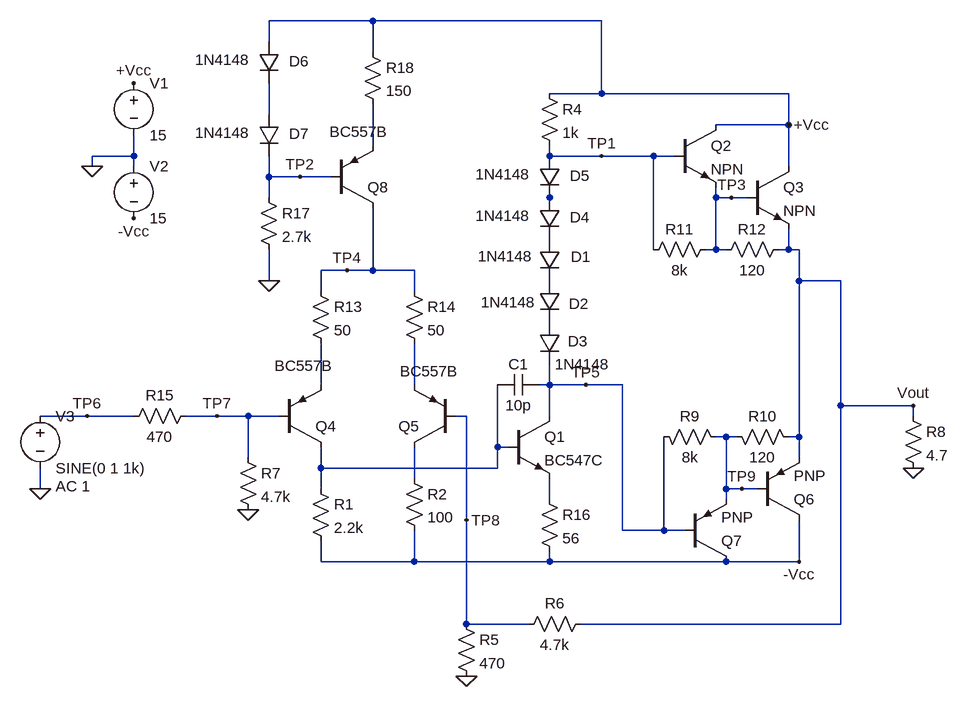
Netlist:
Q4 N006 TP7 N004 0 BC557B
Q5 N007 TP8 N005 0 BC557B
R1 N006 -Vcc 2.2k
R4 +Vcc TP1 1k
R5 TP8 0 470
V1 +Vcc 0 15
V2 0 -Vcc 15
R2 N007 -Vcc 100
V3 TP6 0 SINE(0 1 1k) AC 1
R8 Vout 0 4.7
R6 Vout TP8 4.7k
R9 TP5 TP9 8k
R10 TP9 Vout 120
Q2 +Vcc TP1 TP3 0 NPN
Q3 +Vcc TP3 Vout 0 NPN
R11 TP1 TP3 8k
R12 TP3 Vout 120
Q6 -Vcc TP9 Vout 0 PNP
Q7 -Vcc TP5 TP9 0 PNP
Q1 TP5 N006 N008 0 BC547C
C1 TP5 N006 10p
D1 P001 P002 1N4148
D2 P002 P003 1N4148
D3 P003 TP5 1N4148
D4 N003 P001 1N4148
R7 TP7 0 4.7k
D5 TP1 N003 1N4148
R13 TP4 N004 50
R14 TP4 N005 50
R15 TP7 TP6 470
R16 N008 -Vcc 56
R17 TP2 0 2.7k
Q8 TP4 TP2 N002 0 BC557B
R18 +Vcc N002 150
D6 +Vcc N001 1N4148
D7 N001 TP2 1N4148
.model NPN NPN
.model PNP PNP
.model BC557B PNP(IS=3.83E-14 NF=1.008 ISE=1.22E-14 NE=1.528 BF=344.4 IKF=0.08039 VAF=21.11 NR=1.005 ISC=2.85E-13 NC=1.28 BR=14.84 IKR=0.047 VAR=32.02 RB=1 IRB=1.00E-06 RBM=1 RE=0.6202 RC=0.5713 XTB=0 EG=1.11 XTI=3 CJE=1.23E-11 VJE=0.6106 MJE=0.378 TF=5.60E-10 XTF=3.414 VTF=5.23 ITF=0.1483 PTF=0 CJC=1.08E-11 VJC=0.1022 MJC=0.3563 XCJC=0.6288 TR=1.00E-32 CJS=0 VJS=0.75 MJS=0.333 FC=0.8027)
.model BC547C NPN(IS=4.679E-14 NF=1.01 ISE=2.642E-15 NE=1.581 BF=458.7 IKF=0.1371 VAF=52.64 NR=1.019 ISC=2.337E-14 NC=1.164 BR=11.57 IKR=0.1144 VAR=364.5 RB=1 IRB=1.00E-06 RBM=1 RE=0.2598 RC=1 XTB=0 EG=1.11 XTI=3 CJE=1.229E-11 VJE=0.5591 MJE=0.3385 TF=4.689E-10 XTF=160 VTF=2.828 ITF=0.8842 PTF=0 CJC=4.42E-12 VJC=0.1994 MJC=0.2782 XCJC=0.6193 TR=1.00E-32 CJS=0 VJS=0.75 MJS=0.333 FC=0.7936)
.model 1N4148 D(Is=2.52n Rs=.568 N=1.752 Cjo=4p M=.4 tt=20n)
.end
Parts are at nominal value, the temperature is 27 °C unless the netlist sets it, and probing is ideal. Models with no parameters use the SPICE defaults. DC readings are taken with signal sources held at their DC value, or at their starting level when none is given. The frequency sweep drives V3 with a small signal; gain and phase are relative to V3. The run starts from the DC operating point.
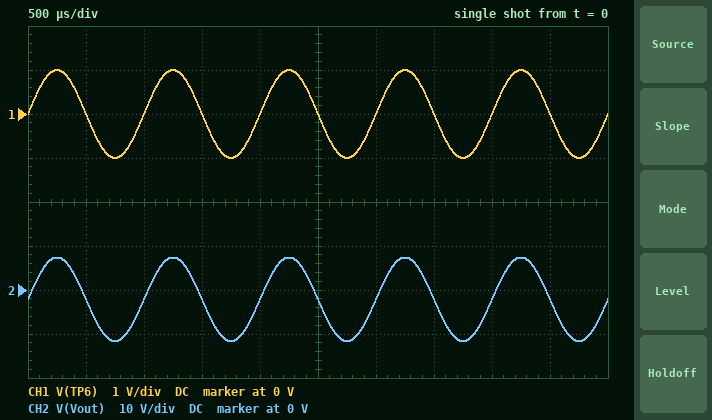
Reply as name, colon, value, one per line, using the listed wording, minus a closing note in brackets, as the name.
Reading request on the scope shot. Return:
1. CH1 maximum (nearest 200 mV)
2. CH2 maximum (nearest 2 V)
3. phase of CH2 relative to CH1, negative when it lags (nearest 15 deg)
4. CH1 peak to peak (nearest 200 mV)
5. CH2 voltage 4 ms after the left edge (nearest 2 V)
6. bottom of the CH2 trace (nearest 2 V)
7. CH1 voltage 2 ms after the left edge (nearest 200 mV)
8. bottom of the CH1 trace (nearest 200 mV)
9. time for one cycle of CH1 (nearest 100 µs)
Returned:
CH1 maximum: 1.0 V
CH2 maximum: 8 V
phase of CH2 relative to CH1, negative when it lags: 0 deg
CH1 peak to peak: 2.0 V
CH2 voltage 4 ms after the left edge: -2 V
bottom of the CH2 trace: -12 V
CH1 voltage 2 ms after the left edge: 0 V
bottom of the CH1 trace: -1.0 V
time for one cycle of CH1: 1.0 ms
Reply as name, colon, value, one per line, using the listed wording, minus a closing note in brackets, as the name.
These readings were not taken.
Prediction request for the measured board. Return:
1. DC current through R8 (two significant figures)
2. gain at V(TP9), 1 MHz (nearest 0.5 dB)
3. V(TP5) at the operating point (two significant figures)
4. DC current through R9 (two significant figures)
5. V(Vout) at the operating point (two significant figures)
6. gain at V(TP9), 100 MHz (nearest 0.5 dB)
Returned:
DC current through R8: 450 mA
gain at V(TP9), 1 MHz: 19.5 dB
V(TP5) at the operating point: -3.9 V
DC current through R9: 110 µA
V(Vout) at the operating point: -2.1 V
gain at V(TP9), 100 MHz: -14.5 dB
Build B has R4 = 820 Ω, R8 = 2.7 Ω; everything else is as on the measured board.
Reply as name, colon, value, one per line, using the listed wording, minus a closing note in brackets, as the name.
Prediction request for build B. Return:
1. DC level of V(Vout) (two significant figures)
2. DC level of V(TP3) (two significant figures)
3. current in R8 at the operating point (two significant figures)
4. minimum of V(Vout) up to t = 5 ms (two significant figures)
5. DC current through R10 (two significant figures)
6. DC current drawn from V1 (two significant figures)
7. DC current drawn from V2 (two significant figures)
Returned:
DC level of V(Vout): -2.0 V
DC level of V(TP3): -1.0 V
current in R8 at the operating point: 730 mA
minimum of V(Vout) up to t = 5 ms: -11 V
DC current through R10: 8.1 mA
DC current drawn from V1: 1.1 A
DC current drawn from V2: 1.8 A
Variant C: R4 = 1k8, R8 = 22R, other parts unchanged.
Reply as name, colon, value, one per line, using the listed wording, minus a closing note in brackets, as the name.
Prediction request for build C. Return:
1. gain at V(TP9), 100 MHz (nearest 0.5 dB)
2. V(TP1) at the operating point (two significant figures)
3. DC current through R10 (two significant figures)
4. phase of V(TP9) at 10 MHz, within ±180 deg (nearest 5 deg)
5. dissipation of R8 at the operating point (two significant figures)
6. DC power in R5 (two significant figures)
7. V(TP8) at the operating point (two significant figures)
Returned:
gain at V(TP9), 100 MHz: -15.0 dB
V(TP1) at the operating point: -750 mV
DC current through R10: 7.5 mA
phase of V(TP9) at 10 MHz, within ±180 deg: -90 deg
dissipation of R8 at the operating point: 270 mW
DC power in R5: 100 µW
V(TP8) at the operating point: -220 mV
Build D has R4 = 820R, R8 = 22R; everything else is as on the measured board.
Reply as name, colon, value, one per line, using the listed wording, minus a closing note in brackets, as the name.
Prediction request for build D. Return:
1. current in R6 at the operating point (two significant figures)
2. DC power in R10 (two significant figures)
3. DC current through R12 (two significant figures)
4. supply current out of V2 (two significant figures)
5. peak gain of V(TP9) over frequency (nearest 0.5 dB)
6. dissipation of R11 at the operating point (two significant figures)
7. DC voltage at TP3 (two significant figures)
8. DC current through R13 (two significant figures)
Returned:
current in R6 at the operating point: 380 µA
DC power in R10: 7.7 mW
DC current through R12: 8.0 mA
supply current out of V2: 1.5 A
peak gain of V(TP9) over frequency: 19.5 dB
dissipation of R11 at the operating point: 91 µW
DC voltage at TP3: -1.0 V
DC current through R13: 830 µA
